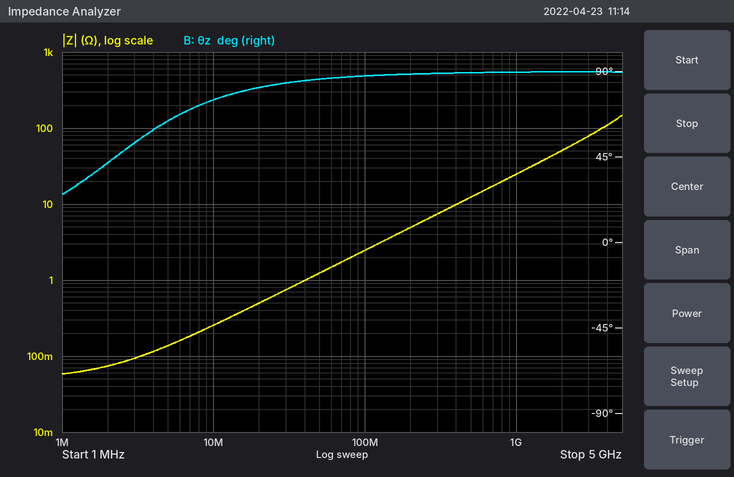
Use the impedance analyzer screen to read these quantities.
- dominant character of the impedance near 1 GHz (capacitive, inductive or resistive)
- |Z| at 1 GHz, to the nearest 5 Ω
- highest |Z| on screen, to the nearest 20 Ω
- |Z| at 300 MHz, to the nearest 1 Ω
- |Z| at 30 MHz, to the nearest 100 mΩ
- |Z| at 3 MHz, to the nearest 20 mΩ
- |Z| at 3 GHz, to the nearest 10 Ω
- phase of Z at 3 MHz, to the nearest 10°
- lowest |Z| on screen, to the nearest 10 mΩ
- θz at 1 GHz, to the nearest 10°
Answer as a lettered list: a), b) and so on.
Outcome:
a) inductive
b) 25 Ω
c) 140 Ω
d) 7 Ω
e) 700 mΩ
f) 100 mΩ
g) 80 Ω
h) 50°
i) 60 mΩ
j) 90°
